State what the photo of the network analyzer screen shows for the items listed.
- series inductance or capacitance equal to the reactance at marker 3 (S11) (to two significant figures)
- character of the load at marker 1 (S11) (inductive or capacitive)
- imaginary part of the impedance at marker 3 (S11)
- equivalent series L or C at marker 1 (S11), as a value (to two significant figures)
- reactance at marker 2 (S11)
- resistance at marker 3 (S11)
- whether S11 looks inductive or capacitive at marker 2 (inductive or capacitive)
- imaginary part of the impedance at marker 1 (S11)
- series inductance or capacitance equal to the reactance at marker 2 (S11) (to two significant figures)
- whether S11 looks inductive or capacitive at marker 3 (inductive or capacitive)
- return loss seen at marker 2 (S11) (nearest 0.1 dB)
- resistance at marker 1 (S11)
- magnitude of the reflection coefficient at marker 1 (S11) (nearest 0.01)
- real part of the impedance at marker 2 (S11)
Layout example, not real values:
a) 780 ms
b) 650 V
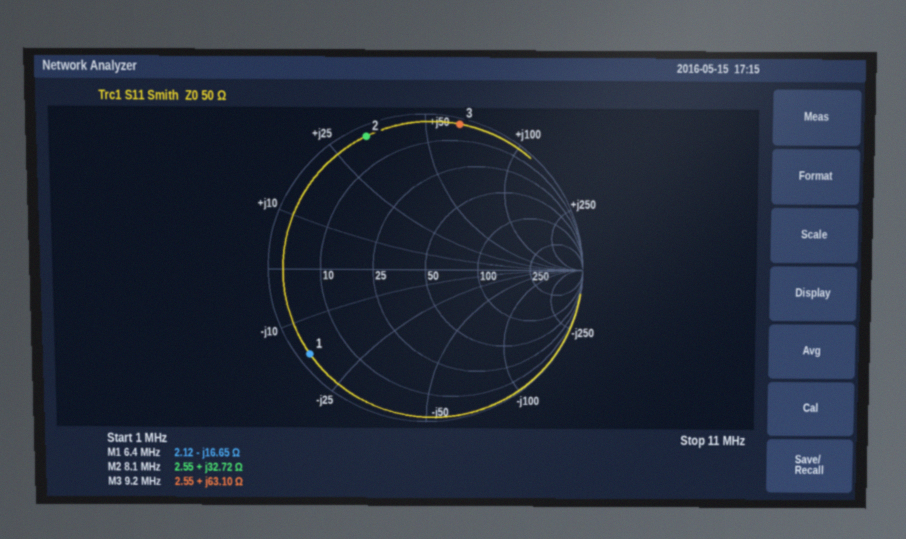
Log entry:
a) 1.1 µH
b) capacitive
c) +63.10 Ω
d) 1.5 nF
e) +32.72 Ω
f) 2.55 Ω
g) inductive
h) -16.65 Ω
i) 640 nH
j) inductive
k) 0.6 dB
l) 2.12 Ω
m) 0.93
n) 2.55 Ω
